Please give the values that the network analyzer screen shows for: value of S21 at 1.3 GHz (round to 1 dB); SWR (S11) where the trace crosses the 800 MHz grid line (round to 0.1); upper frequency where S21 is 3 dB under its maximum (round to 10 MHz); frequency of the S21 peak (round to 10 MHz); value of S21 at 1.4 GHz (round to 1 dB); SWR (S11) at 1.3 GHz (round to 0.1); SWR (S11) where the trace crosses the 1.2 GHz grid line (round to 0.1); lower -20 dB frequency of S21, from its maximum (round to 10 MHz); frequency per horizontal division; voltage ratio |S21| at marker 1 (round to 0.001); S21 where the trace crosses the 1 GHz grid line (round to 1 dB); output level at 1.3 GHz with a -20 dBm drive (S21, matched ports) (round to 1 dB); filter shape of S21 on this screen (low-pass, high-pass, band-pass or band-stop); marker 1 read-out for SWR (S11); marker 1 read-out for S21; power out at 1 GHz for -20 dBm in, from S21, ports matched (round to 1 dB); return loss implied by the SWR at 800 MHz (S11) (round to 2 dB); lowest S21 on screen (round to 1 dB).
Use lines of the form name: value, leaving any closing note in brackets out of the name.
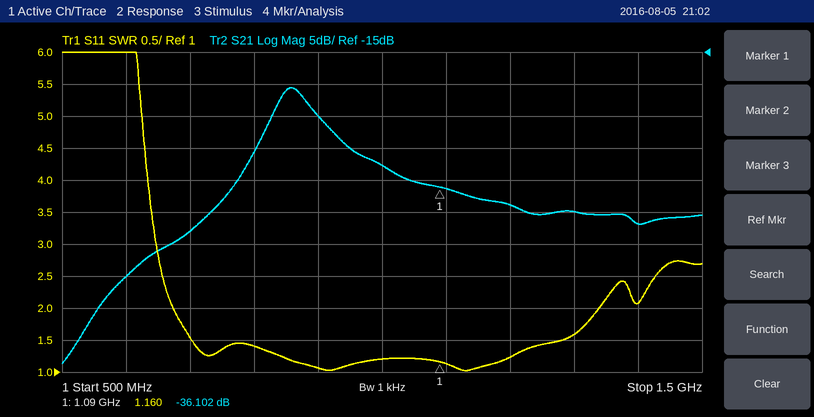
value of S21 at 1.3 GHz: -40 dB
SWR (S11) where the trace crosses the 800 MHz grid line: 1.4
upper frequency where S21 is 3 dB under its maximum: 890 MHz
frequency of the S21 peak: 860 MHz
value of S21 at 1.4 GHz: -42 dB
SWR (S11) at 1.3 GHz: 1.6
SWR (S11) where the trace crosses the 1.2 GHz grid line: 1.2
lower -20 dB frequency of S21, from its maximum: 730 MHz
frequency per horizontal division: 100 MHz
voltage ratio |S21| at marker 1: 0.016
S21 where the trace crosses the 1 GHz grid line: -33 dB
output level at 1.3 GHz with a -20 dBm drive (S21, matched ports): -60 dBm
filter shape of S21 on this screen: band-pass
marker 1 read-out for SWR: 1.160
marker 1 read-out for S21: -36.102 dB
power out at 1 GHz for -20 dBm in, from S21, ports matched: -53 dBm
return loss implied by the SWR at 800 MHz (S11): 16 dB
lowest S21 on screen: -64 dB
